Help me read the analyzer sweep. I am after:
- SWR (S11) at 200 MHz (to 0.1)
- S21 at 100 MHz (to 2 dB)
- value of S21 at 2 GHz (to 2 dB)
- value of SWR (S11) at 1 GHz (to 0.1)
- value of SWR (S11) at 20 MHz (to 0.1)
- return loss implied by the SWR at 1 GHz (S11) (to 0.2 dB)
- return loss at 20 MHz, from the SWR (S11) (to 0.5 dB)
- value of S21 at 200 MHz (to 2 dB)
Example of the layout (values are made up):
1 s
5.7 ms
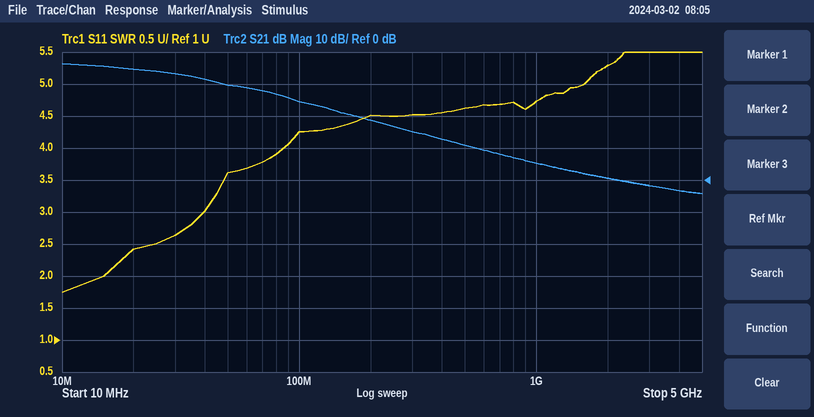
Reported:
4.5
24 dB
0 dB
4.7
2.4
3.8 dB
7.5 dB
18 dB
